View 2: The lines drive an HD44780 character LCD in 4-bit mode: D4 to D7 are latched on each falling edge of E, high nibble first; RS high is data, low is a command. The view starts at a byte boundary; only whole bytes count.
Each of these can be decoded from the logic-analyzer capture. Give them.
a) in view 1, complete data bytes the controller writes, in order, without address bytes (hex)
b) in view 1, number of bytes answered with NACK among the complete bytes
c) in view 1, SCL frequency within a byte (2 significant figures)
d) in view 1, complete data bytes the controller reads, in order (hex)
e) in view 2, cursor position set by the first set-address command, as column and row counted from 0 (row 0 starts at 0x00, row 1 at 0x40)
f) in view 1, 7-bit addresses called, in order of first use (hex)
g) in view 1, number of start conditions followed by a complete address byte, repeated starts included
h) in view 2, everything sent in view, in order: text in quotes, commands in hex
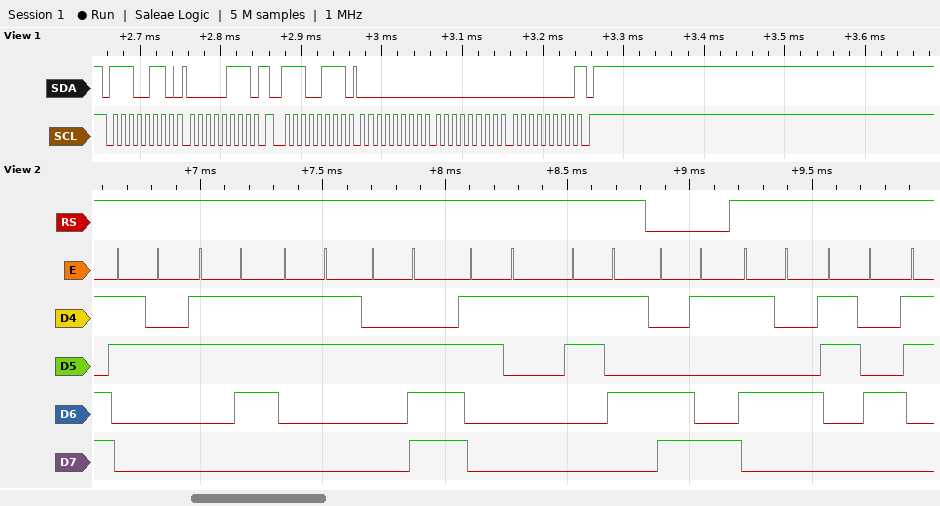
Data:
07
1
100 kHz
00 00 00
column 9, row 1
0x73
2
"273.15" 0xC9 "T4"
